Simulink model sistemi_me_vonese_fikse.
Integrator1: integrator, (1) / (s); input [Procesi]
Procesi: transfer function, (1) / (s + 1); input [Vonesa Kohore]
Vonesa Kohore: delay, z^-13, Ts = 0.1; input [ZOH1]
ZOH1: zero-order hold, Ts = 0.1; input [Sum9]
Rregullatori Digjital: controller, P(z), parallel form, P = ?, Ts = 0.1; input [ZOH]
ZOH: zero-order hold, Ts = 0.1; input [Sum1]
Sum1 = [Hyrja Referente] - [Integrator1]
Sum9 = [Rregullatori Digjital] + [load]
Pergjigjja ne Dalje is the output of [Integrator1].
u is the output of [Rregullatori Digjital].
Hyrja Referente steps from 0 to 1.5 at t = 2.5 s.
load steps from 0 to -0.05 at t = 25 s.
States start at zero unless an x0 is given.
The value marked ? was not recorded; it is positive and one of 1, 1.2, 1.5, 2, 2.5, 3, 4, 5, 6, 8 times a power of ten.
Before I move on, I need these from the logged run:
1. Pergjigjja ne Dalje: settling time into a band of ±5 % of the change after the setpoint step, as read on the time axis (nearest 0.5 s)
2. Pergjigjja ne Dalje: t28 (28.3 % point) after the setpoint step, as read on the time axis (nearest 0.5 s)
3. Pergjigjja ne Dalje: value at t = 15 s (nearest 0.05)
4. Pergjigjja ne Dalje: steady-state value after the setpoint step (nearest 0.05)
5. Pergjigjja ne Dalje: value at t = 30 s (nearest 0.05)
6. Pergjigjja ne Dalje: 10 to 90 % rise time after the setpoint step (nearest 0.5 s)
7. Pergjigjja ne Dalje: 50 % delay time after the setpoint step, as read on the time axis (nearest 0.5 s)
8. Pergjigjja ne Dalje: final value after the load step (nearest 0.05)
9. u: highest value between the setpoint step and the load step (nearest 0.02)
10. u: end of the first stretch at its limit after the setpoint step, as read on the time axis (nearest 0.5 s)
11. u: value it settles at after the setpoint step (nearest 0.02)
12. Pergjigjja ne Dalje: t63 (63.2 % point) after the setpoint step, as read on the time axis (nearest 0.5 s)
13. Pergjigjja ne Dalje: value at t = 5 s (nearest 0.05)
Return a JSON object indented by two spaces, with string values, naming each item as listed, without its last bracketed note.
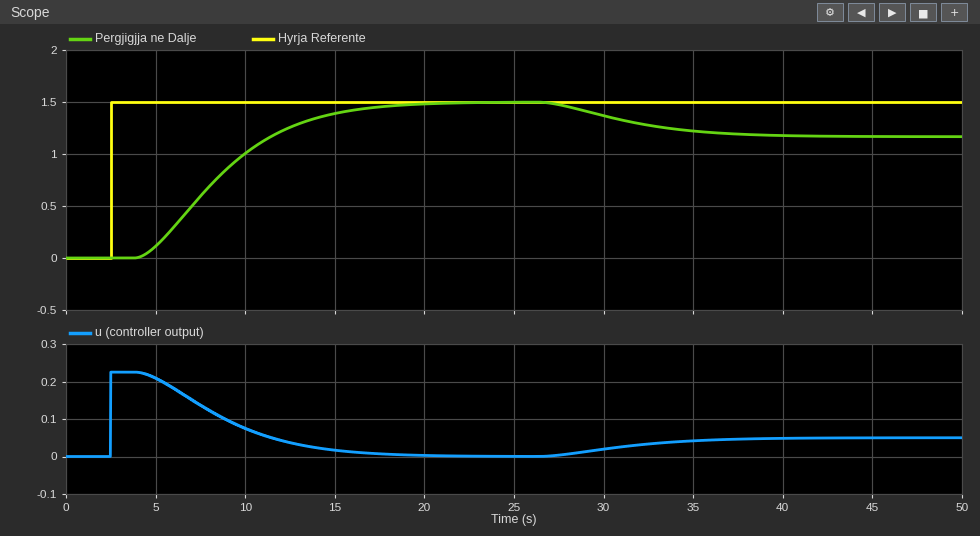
{
  "Pergjigjja ne Dalje: settling time into a band of ±5 % of the change after the setpoint step, as read on the time axis": "16.0 s",
  "Pergjigjja ne Dalje: t28 (28.3 % point) after the setpoint step, as read on the time axis": "6.5 s",
  "Pergjigjja ne Dalje: value at t = 15 s": "1.40",
  "Pergjigjja ne Dalje: steady-state value after the setpoint step": "1.50",
  "Pergjigjja ne Dalje: value at t = 30 s": "1.35",
  "Pergjigjja ne Dalje: 10 to 90 % rise time after the setpoint step": "9.0 s",
  "Pergjigjja ne Dalje: 50 % delay time after the setpoint step, as read on the time axis": "8.5 s",
  "Pergjigjja ne Dalje: final value after the load step": "1.15",
  "u: highest value between the setpoint step and the load step": "0.22",
  "u: end of the first stretch at its limit after the setpoint step, as read on the time axis": "4.5 s",
  "u: value it settles at after the setpoint step": "0.00",
  "Pergjigjja ne Dalje: t63 (63.2 % point) after the setpoint step, as read on the time axis": "9.5 s",
  "Pergjigjja ne Dalje: value at t = 5 s": "0.10"
}
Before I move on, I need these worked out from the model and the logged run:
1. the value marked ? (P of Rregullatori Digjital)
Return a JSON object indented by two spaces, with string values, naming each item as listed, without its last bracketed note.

{
  "the value marked ?": "0.15"
}
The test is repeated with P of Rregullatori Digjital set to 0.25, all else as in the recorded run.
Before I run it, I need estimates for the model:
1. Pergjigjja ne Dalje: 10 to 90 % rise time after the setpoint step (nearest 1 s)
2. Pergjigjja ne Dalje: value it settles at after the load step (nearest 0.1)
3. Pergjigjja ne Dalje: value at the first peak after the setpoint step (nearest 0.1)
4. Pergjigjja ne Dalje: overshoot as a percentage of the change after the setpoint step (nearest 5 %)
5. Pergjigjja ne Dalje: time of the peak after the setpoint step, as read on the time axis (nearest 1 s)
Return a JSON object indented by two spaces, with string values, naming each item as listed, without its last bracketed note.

{
  "Pergjigjja ne Dalje: 10 to 90 % rise time after the setpoint step": "4 s",
  "Pergjigjja ne Dalje: value it settles at after the load step": "1.3",
  "Pergjigjja ne Dalje: value at the first peak after the setpoint step": "1.6",
  "Pergjigjja ne Dalje: overshoot as a percentage of the change after the setpoint step": "10 %",
  "Pergjigjja ne Dalje: time of the peak after the setpoint step, as read on the time axis": "13 s"
}
